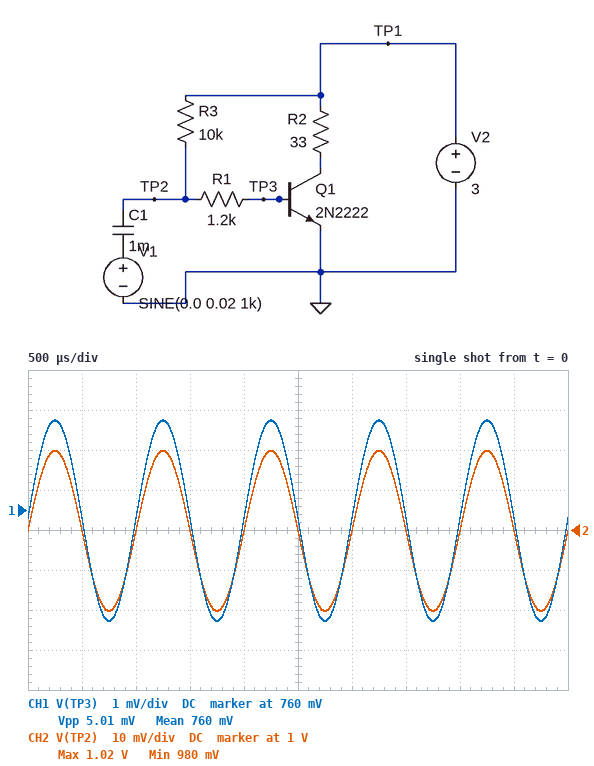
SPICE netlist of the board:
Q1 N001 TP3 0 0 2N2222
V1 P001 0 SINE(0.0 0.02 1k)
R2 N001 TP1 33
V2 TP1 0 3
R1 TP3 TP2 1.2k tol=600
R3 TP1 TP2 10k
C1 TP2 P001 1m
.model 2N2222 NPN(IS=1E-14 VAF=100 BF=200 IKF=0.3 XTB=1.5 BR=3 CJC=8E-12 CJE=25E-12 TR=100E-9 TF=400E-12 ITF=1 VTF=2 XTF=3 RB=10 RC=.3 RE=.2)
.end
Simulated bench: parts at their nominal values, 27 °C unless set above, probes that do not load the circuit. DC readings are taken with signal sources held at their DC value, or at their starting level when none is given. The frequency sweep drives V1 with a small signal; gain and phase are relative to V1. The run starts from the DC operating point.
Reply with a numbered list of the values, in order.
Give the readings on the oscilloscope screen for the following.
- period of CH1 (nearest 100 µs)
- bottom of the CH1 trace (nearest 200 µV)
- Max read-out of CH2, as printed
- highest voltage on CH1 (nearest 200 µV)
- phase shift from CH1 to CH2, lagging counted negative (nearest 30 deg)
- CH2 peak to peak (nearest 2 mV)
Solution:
1. 1.0 ms
2. 757.2 mV
3. 1.02 V
4. 762.2 mV
5. 0 deg
6. 40 mV
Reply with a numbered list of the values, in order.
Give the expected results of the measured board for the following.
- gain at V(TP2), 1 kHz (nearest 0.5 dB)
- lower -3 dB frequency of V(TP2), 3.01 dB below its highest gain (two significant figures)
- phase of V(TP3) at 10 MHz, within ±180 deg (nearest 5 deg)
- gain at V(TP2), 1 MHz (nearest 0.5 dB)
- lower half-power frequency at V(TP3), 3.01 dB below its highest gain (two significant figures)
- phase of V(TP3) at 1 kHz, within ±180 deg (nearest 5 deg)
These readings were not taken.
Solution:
1. 0 dB
2. 130 mHz
3. -60 deg
4. 0 dB
5. 130 mHz
6. 0 deg
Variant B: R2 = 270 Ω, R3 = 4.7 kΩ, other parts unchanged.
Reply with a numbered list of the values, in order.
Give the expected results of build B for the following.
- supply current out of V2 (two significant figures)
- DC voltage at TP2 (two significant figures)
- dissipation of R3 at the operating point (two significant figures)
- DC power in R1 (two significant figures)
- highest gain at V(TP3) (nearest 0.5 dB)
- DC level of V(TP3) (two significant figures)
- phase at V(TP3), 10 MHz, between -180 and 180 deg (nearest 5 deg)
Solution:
1. 11 mA
2. 1.2 V
3. 700 µW
4. 180 µW
5. -36.0 dB
6. 730 mV
7. 0 deg
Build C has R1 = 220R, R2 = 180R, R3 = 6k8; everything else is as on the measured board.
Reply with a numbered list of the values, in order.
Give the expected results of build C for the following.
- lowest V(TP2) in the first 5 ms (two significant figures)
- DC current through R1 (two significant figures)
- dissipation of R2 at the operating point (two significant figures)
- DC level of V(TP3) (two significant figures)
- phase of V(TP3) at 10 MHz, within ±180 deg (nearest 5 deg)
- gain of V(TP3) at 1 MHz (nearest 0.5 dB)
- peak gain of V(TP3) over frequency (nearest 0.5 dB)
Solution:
1. 790 mV
2. 320 µA
3. 47 mW
4. 740 mV
5. 0 deg
6. -25.0 dB
7. -23.0 dB
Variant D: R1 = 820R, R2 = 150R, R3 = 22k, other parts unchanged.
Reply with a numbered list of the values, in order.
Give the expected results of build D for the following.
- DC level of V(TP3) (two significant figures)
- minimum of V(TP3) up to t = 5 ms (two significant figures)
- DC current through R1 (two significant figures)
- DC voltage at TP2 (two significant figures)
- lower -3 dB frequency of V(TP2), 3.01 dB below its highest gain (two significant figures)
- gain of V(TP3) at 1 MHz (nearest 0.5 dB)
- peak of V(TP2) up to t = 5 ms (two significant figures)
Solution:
1. 740 mV
2. 730 mV
3. 99 µA
4. 820 mV
5. 170 mHz
6. -21.5 dB
7. 840 mV
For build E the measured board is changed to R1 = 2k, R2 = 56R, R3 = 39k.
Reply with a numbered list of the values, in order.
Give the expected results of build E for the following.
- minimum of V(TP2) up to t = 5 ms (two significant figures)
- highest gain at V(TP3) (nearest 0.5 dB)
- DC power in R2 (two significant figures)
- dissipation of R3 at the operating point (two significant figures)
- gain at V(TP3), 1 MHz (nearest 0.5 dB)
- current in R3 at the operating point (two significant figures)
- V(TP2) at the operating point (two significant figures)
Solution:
1. 810 mV
2. -14.0 dB
3. 6.7 mW
4. 120 µW
5. -16.0 dB
6. 56 µA
7. 830 mV
